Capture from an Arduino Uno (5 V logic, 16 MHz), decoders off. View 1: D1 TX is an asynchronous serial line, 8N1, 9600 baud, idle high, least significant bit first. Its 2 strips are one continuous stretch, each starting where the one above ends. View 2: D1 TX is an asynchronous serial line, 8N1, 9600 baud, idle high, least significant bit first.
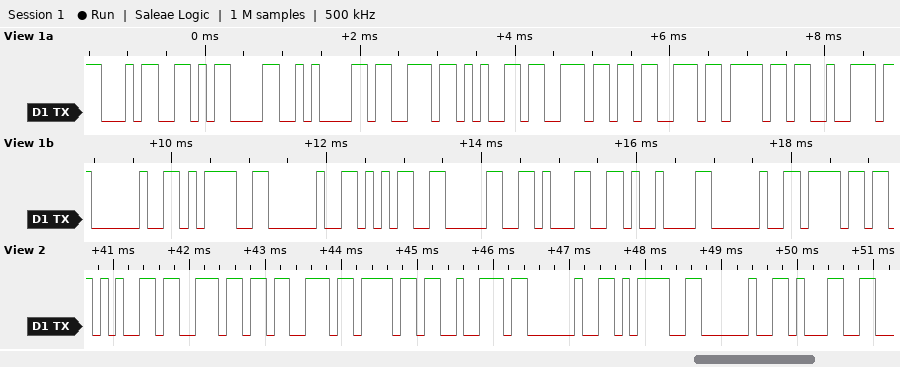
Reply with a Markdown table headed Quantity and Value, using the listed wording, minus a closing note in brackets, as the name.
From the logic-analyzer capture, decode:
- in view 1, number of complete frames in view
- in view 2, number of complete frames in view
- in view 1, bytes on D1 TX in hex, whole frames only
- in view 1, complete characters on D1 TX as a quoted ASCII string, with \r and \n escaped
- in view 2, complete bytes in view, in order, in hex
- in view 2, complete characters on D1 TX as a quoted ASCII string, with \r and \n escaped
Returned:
| Quantity | Value |
|---|---|
| in view 1, number of complete frames in view | 18 |
| in view 2, number of complete frames in view | 9 |
| in view 1, bytes on D1 TX in hex, whole frames only | 34 0D 0A 73 65 6E 73 6F 72 20 3D 20 35 30 31 09 20 6F |
| in view 1, complete characters on D1 TX as a quoted ASCII string, with \r and \n escaped | "4\r\nsensor = 501\t o" |
| in view 2, complete bytes in view, in order, in hex | 65 6E 73 6F 72 20 3D 20 31 |
| in view 2, complete characters on D1 TX as a quoted ASCII string, with \r and \n escaped | "ensor = 1" |
